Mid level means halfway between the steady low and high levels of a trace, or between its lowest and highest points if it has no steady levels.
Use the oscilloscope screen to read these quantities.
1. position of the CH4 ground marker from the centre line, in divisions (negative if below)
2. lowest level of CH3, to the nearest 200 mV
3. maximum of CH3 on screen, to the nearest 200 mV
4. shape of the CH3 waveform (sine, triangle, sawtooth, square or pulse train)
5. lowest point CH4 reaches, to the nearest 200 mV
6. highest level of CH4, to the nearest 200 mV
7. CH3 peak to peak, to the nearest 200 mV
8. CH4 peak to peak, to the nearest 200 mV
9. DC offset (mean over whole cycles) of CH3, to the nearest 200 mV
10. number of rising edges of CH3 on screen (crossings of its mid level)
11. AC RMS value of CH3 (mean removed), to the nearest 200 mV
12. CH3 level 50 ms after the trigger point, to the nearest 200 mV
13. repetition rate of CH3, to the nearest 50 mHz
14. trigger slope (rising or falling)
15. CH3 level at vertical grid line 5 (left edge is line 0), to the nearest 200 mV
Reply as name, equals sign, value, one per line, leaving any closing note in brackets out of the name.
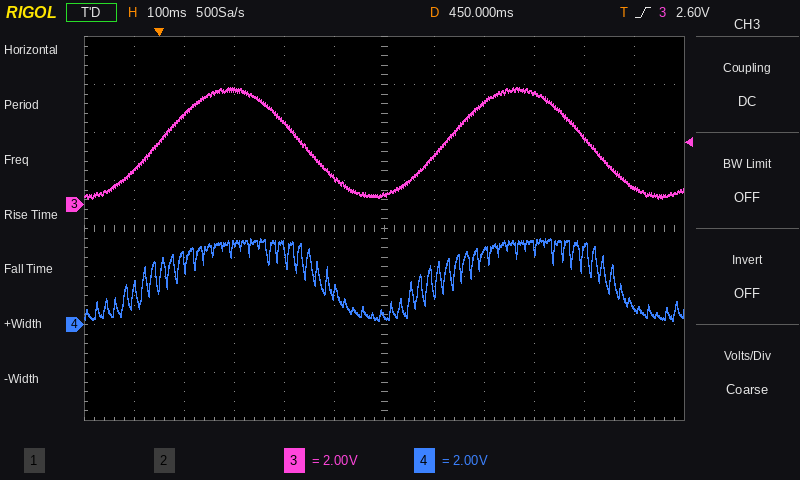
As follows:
position of the CH4 ground marker from the centre line, in divisions = -2.0 div
lowest level of CH3, to the nearest 200 mV = 200 mV
maximum of CH3 on screen, to the nearest 200 mV = 4.8 V
shape of the CH3 waveform = sine
lowest point CH4 reaches, to the nearest 200 mV = 200 mV
highest level of CH4, to the nearest 200 mV = 3.6 V
CH3 peak to peak, to the nearest 200 mV = 4.6 V
CH4 peak to peak, to the nearest 200 mV = 3.4 V
DC offset (mean over whole cycles) of CH3, to the nearest 200 mV = 2.6 V
number of rising edges of CH3 on screen = 2
AC RMS value of CH3 (mean removed), to the nearest 200 mV = 1.6 V
CH3 level 50 ms after the trigger point, to the nearest 200 mV = 3.8 V
repetition rate of CH3, to the nearest 50 mHz = 1.75 Hz
trigger slope = rising
CH3 level at vertical grid line 5 (left edge is line 0), to the nearest 200 mV = 1.2 V
